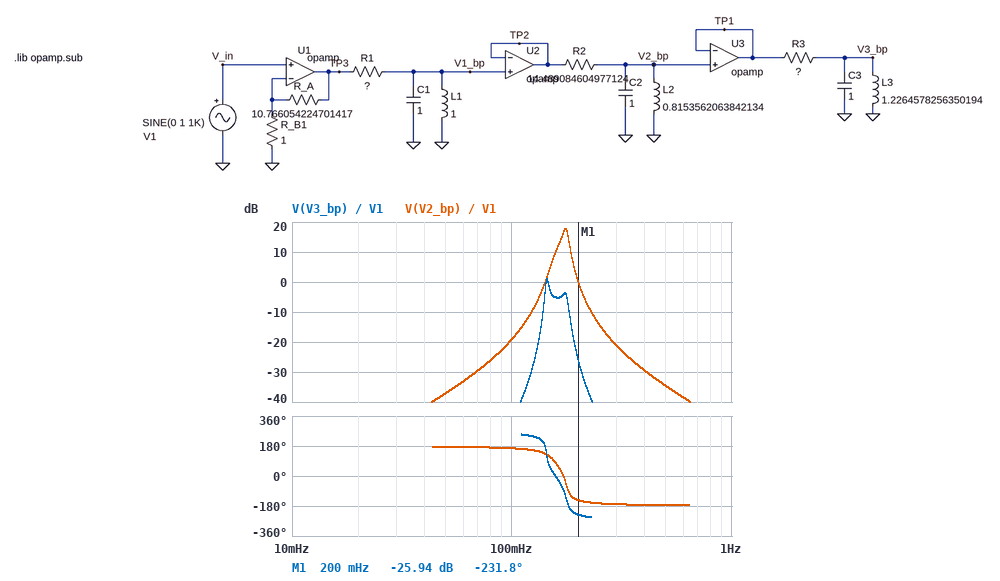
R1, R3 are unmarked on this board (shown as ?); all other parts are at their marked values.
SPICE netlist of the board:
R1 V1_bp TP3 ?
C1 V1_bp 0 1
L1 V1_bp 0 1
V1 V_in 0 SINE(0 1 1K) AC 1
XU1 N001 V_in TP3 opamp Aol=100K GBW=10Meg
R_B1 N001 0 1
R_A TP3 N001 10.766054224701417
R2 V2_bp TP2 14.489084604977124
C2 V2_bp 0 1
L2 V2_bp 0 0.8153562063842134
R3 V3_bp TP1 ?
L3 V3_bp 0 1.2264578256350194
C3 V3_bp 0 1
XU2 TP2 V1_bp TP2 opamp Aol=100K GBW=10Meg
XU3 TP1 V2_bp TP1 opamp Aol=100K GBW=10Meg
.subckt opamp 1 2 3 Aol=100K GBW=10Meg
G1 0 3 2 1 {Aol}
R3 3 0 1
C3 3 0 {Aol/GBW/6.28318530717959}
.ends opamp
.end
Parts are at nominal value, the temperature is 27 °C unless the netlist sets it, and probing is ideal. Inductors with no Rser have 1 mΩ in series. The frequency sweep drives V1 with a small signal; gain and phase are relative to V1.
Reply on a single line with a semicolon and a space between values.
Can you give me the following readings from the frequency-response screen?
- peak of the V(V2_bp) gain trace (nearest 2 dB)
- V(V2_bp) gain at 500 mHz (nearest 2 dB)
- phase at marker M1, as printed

18 dB; -34 dB; -231.8 deg
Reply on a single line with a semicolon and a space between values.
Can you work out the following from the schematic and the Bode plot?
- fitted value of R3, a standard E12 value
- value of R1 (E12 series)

33 Ω; 5.6 Ω
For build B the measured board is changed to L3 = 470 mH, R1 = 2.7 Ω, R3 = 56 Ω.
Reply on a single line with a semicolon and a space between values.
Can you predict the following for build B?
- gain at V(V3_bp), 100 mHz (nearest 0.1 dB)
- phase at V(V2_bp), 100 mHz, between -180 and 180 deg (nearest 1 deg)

-56.9 dB; 156 deg
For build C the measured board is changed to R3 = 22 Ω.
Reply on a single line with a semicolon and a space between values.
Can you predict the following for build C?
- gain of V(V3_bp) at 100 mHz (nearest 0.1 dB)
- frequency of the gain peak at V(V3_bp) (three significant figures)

-42.4 dB; 145 mHz
